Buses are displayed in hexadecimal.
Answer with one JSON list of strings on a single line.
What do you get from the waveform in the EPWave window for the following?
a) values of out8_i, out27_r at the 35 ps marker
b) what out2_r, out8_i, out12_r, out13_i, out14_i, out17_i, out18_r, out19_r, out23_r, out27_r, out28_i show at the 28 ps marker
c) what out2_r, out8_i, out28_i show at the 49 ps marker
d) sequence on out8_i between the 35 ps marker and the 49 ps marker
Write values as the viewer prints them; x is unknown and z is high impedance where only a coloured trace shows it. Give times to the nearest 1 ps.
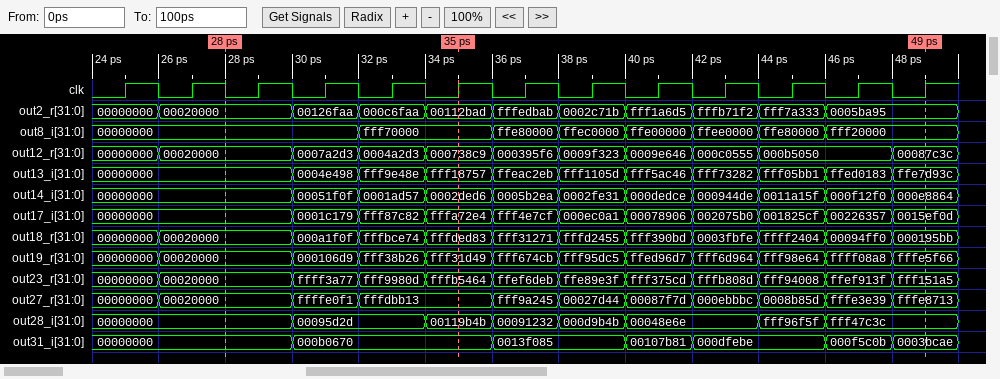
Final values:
["out8_i=fff70000, out27_r=fffdbb13", "out2_r=00020000, out8_i=00000000, out12_r=00020000, out13_i=00000000, out14_i=00000000, out17_i=00000000, out18_r=00020000, out19_r=00020000, out23_r=00020000, out27_r=00020000, out28_i=00000000", "out2_r=0005ba95, out8_i=fff20000, out28_i=fff47c3c", "fff70000, ffe80000, ffec0000, ffe00000, ffee0000, ffe80000, fff20000"]
